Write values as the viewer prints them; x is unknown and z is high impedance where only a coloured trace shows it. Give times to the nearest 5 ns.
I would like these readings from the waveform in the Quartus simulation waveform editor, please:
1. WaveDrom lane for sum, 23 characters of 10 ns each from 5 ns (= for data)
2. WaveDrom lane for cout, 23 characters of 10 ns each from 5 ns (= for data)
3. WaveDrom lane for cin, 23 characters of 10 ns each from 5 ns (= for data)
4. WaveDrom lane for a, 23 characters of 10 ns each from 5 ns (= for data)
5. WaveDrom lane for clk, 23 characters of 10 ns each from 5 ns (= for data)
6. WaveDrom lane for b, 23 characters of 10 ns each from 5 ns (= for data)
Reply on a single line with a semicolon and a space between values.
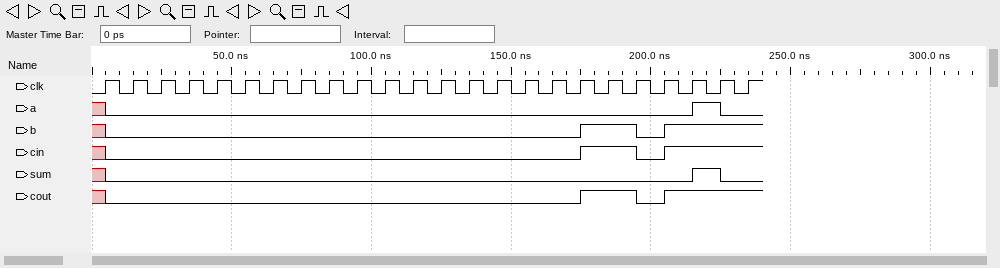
{name: 'sum', wave: '0....................10'}; {name: 'cout', wave: '0................1.01..'}; {name: 'cin', wave: '0................1.01..'}; {name: 'a', wave: '0....................10'}; {name: 'clk', wave: 'p......................'}; {name: 'b', wave: '0................1.01..'}
